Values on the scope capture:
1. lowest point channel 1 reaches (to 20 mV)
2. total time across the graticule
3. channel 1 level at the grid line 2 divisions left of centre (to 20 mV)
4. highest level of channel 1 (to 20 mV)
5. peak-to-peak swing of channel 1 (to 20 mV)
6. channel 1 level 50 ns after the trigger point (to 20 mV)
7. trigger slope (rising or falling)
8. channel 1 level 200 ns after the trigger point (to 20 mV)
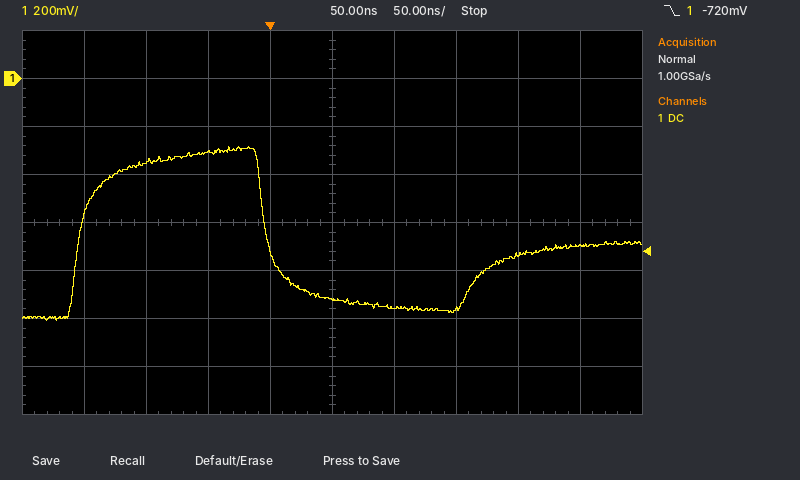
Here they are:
-1.00 V
500 ns
-300 mV
-280 mV
720 mV
-920 mV
falling
-740 mV
